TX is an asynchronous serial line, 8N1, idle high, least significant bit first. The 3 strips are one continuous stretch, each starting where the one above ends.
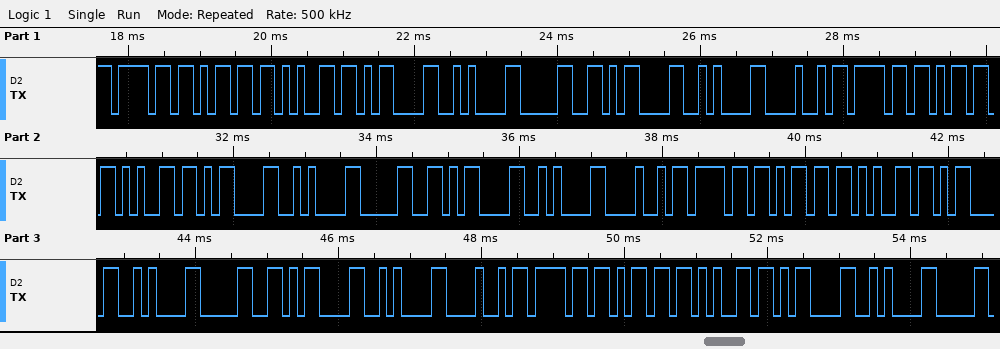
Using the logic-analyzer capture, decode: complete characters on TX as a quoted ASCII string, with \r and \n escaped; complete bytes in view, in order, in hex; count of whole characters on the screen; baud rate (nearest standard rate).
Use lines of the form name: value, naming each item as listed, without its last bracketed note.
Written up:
complete characters on TX as a quoted ASCII string, with \r and \n escaped: "ome\r\n0\r\nHome\r\n0\r\nHome\r\n0\r\nHome\r\n"
complete bytes in view, in order, in hex: 6F 6D 65 0D 0A 30 0D 0A 48 6F 6D 65 0D 0A 30 0D 0A 48 6F 6D 65 0D 0A 30 0D 0A 48 6F 6D 65 0D 0A
count of whole characters on the screen: 32
baud rate: 9600 baud
